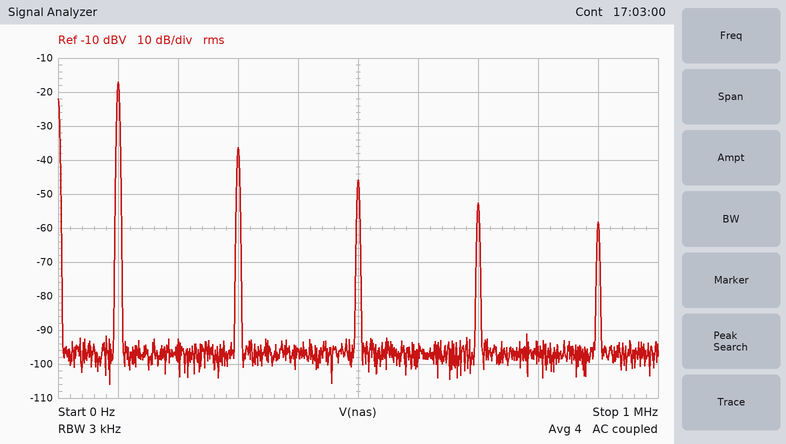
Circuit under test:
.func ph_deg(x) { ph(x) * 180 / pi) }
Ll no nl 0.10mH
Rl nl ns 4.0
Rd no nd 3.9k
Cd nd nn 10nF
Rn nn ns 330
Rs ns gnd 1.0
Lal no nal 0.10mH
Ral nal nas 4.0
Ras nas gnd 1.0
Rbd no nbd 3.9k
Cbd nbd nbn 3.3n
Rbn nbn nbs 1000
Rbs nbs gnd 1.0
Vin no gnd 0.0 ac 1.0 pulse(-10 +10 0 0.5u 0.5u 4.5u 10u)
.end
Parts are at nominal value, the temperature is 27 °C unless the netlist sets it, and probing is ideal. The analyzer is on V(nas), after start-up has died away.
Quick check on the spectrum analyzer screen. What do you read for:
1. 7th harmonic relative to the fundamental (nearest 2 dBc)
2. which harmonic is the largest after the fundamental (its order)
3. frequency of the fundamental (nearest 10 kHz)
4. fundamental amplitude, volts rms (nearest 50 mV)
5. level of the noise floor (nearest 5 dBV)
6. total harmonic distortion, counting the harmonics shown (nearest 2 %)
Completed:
-36 dBc
3
100 kHz
150 mV
-95 dBV
12 %
